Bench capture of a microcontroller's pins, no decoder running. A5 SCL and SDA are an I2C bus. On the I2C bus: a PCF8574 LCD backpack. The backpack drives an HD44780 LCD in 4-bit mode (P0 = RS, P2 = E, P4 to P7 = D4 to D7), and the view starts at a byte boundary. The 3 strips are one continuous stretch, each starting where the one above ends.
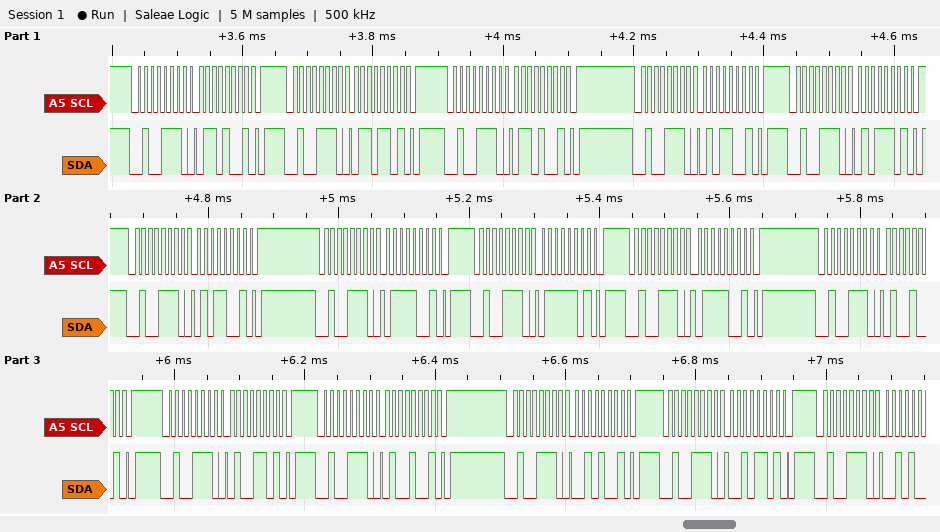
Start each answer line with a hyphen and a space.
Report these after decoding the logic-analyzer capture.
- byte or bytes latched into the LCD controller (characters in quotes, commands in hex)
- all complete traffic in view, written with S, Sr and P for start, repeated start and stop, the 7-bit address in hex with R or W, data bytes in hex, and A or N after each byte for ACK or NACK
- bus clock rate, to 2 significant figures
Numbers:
- 'e' 't'
- S 27W A 69 A P S 27W A 6D A P S 27W A 69 A P S 27W A 59 A P S 27W A 5D A P S 27W A 59 A P S 27W A 79 A P S 27W A 7D A P S 27W A 79 A P S 27W A 49 A P S 27W A 4D A P S 27W A 49 A P S 27W A 29 A P S 27W A 2D A P S 27W A
- 100 kHz
